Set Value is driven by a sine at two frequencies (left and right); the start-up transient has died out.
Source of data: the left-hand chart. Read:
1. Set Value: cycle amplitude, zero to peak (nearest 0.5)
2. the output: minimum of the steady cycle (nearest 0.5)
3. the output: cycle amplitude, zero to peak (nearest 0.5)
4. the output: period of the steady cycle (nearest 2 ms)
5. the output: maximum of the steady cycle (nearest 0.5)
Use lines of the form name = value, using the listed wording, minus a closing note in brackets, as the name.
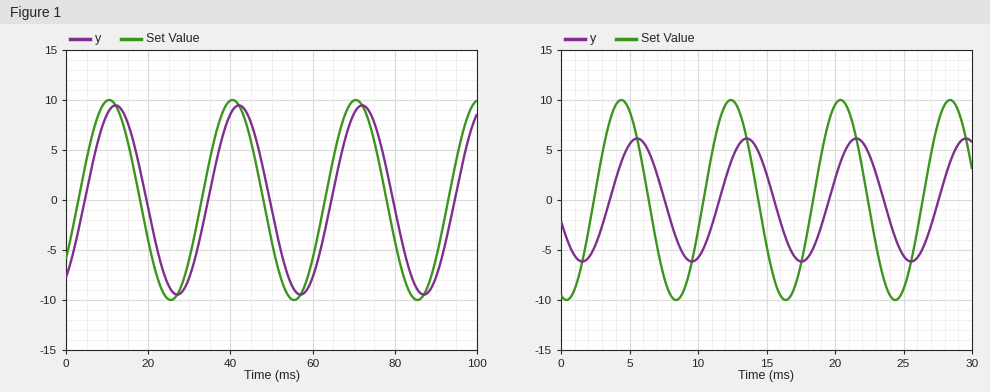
Set Value: cycle amplitude, zero to peak = 10.0
the output: minimum of the steady cycle = -9.5
the output: cycle amplitude, zero to peak = 9.5
the output: period of the steady cycle = 30 ms
the output: maximum of the steady cycle = 9.5
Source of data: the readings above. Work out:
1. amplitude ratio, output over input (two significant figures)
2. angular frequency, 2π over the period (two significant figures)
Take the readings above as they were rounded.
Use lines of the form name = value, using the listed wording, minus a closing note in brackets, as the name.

amplitude ratio, output over input = 0.95
angular frequency, 2π over the period = 0.21 rad/ms
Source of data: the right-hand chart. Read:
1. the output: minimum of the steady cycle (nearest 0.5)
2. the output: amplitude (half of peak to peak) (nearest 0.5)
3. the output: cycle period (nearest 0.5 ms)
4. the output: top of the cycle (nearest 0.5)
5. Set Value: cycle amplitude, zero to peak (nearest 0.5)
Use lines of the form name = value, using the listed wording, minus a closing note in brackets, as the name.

the output: minimum of the steady cycle = -6.0
the output: amplitude (half of peak to peak) = 6.0
the output: cycle period = 8.0 ms
the output: top of the cycle = 6.0
Set Value: cycle amplitude, zero to peak = 10.0
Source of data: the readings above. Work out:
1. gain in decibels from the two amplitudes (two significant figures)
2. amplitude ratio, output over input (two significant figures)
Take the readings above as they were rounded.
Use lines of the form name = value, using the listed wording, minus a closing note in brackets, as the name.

gain in decibels from the two amplitudes = -4.4 dB
amplitude ratio, output over input = 0.60
